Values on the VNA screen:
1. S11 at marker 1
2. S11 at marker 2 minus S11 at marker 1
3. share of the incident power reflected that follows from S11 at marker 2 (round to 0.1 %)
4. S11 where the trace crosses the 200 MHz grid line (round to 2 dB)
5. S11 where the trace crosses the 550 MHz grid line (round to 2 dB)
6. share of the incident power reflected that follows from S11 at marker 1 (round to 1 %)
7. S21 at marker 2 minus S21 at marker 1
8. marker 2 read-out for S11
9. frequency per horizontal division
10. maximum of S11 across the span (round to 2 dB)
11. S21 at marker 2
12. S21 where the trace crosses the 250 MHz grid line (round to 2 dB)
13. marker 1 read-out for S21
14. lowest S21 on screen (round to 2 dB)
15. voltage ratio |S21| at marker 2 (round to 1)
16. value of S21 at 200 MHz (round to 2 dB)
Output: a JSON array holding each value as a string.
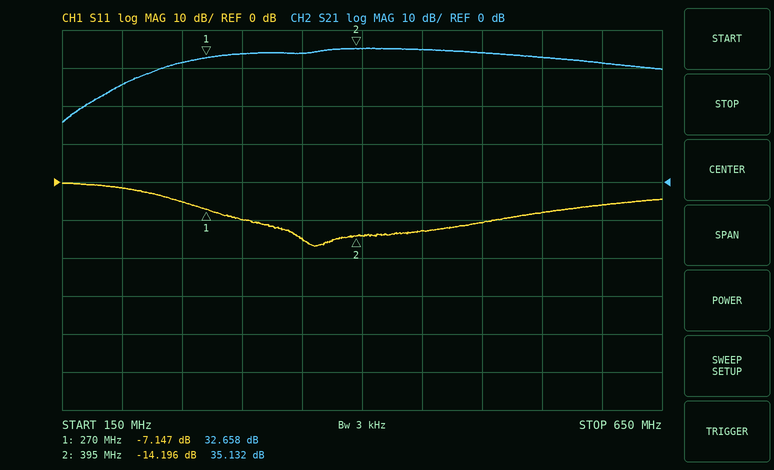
["-7.147 dB", "-7.049 dB", "3.8 %", "-2 dB", "-8 dB", "19 %", "2.474 dB", "-14.196 dB", "50 MHz", "0 dB", "35.132 dB", "32 dB", "32.658 dB", "16 dB", "57", "26 dB"]
